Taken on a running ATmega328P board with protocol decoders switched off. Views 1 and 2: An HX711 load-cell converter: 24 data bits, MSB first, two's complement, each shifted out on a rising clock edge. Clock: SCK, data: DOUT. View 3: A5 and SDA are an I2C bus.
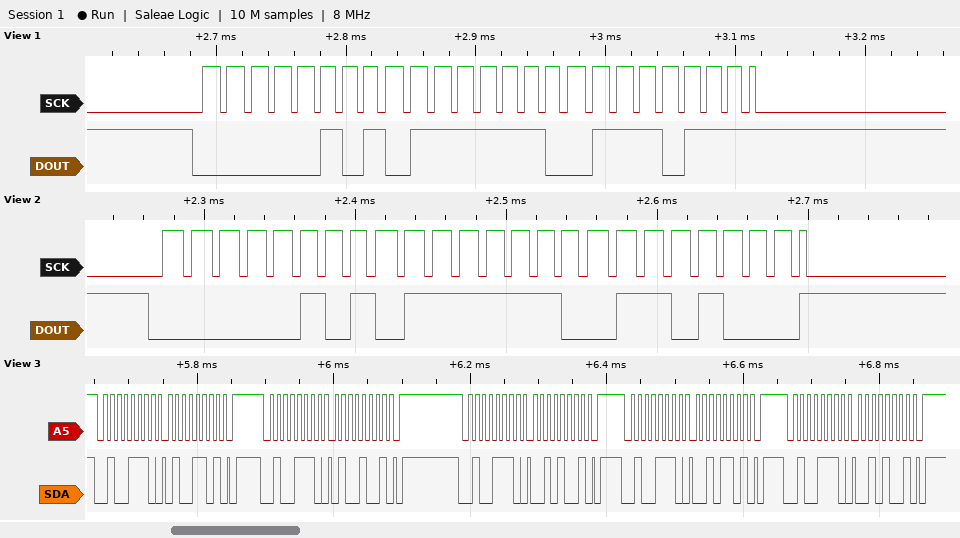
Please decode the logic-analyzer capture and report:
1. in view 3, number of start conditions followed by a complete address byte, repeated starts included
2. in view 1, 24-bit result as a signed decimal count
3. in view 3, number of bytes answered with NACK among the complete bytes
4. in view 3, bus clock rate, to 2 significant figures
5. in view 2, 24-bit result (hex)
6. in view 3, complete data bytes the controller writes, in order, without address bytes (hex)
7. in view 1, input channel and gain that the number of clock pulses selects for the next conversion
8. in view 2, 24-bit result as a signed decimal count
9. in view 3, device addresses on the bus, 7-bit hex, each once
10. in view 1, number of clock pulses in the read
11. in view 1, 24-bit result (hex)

5
360055
0
100 kHz
0x057E68
4D 49 29 2D 29
channel A, gain 128
360040
0x27
25
0x057E77
